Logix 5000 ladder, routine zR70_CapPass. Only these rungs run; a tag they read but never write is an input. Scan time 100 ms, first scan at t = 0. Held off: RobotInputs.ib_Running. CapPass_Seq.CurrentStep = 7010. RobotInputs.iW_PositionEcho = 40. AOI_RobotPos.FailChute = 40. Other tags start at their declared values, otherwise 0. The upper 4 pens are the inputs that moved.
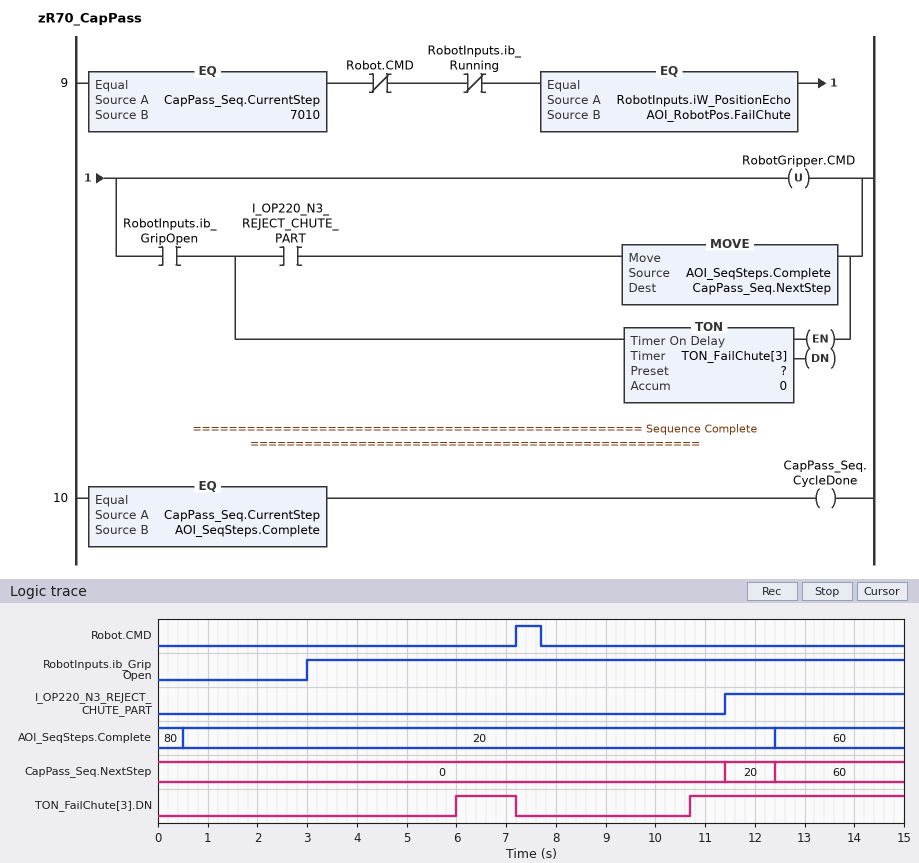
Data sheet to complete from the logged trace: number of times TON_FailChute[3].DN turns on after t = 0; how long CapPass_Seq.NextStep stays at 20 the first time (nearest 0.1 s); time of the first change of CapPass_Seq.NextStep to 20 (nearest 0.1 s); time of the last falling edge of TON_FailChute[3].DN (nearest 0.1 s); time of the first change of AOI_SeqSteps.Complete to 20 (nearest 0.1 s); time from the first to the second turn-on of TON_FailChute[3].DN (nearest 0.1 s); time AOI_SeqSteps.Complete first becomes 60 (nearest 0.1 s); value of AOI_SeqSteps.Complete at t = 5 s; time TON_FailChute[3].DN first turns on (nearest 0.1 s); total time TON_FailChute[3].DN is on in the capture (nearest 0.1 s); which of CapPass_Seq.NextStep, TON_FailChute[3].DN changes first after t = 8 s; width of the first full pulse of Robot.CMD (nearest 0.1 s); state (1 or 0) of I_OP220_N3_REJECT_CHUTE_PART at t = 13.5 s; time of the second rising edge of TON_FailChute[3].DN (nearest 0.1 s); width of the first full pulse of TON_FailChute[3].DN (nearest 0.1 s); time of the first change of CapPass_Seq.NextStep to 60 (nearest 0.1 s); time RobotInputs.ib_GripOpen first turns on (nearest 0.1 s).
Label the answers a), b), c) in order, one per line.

a) 2
b) 1.0 s
c) 11.4 s
d) 7.2 s
e) 0.5 s
f) 4.7 s
g) 12.4 s
h) 20
i) 6.0 s
j) 5.5 s
k) TON_FailChute[3].DN
l) 0.5 s
m) 1
n) 10.7 s
o) 1.2 s
p) 12.4 s
q) 3.0 s
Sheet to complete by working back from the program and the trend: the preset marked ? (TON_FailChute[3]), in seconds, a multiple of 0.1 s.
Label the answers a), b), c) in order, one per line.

a) 3.0 s
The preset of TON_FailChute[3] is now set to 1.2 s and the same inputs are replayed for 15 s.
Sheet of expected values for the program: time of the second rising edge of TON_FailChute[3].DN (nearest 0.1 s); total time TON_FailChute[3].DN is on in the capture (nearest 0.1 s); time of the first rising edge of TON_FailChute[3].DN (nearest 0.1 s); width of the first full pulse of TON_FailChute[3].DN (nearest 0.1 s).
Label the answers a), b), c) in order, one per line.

a) 8.9 s
b) 9.1 s
c) 4.2 s
d) 3.0 s
